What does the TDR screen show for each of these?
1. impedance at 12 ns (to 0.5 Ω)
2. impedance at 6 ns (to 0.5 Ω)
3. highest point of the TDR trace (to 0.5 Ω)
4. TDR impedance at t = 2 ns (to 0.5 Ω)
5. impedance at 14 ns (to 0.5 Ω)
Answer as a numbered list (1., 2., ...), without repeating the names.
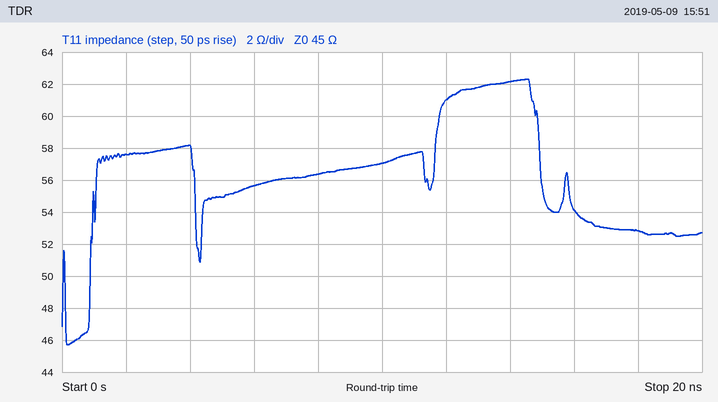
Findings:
1. 61.0 Ω
2. 55.5 Ω
3. 62.5 Ω
4. 57.5 Ω
5. 62.0 Ω
